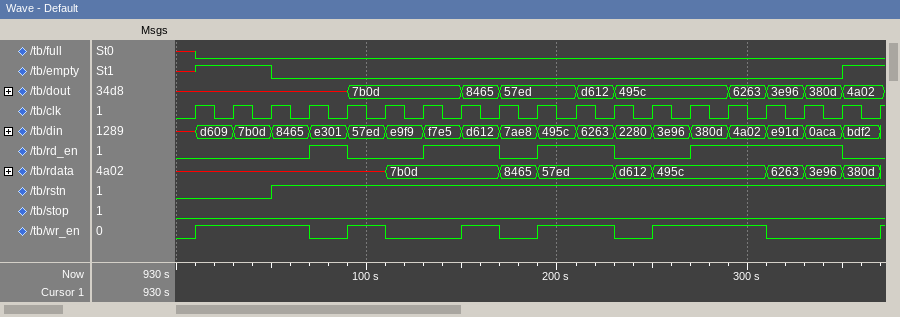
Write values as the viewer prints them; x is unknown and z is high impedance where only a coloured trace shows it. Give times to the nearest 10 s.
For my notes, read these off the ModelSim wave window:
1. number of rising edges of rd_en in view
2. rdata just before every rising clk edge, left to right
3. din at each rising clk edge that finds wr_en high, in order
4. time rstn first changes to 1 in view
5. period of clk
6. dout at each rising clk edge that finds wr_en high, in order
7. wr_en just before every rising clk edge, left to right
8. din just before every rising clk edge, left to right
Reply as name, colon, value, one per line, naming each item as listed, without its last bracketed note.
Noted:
number of rising edges of rd_en in view: 4
rdata just before every rising clk edge, left to right: x, x, x, x, x, x, 7b0d, 7b0d, 7b0d, 8465, 57ed, 57ed, d612, 495c, 495c, 495c, 6263, 3e96, 380d
din at each rising clk edge that finds wr_en high, in order: d609, 7b0d, 8465, 57ed, d612, 495c, 6263, 3e96, 380d, 4a02
time rstn first changes to 1 in view: 50 s
period of clk: 20 s
dout at each rising clk edge that finds wr_en high, in order: x, x, x, 7b0d, 8465, 57ed, d612, 495c, 495c, 6263
wr_en just before every rising clk edge, left to right: 0 1 1 1 0 1 0 0 1 0 1 1 0 1 1 1 0 0 0
din just before every rising clk edge, left to right: x, d609, 7b0d, 8465, e301, 57ed, e9f9, f7e5, d612, 7ae8, 495c, 6263, 2280, 3e96, 380d, 4a02, e91d, 0aca, bdf2
